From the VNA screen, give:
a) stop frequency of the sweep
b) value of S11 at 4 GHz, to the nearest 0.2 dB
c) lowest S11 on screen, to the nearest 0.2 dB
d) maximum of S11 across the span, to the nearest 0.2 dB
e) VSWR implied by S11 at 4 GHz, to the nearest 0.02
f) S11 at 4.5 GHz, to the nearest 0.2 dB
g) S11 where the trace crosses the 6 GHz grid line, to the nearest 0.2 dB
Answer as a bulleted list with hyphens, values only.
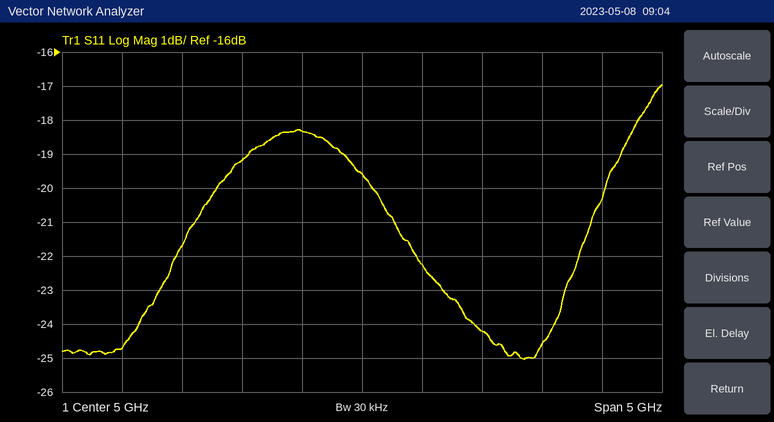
- 7.5 GHz
- -19.2 dB
- -25.0 dB
- -17.0 dB
- 1.24
- -18.4 dB
- -24.2 dB
